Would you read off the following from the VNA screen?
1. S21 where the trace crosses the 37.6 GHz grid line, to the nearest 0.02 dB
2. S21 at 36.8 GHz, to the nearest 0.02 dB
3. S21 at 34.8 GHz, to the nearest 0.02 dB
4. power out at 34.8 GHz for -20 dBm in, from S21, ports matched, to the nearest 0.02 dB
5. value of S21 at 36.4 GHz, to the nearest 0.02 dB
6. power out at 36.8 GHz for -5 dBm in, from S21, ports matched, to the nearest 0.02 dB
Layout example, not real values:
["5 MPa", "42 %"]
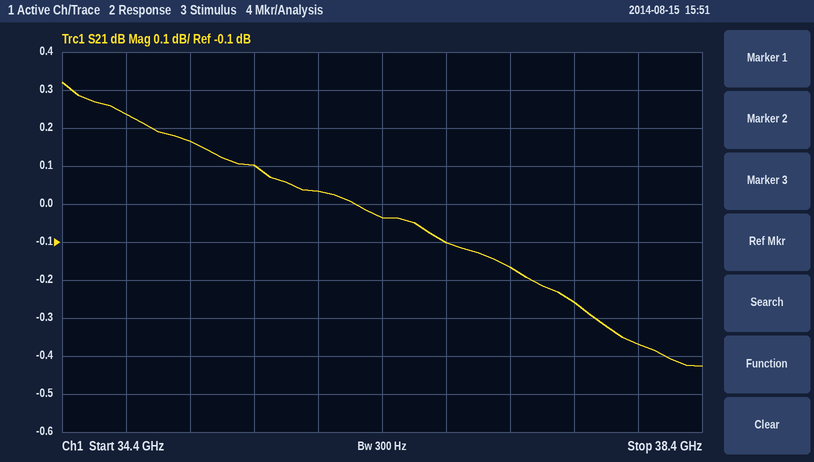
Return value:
["-0.26 dB", "-0.10 dB", "0.24 dB", "-19.76 dBm", "-0.04 dB", "-5.10 dBm"]
